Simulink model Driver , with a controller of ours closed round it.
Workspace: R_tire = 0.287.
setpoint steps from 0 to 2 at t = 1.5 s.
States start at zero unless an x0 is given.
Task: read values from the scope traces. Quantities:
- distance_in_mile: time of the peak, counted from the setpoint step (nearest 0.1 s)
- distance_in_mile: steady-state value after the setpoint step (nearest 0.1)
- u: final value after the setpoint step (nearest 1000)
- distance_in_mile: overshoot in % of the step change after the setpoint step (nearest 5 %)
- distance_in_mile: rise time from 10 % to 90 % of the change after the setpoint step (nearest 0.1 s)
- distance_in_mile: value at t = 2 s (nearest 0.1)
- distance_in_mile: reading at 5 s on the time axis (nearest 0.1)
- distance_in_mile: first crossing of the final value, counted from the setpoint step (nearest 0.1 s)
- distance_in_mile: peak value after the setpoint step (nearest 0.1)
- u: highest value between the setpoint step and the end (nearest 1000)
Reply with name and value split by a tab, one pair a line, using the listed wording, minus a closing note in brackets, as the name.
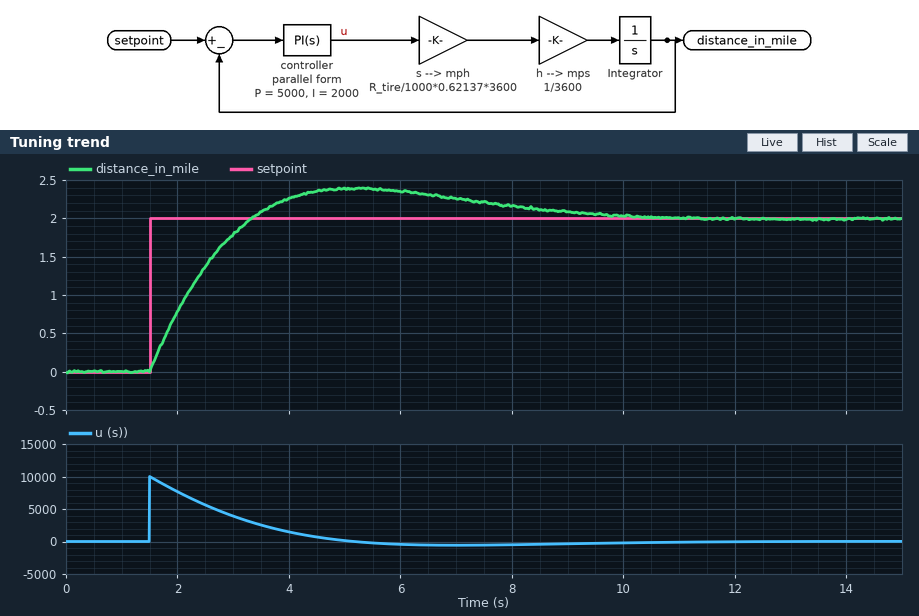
distance_in_mile: time of the peak, counted from the setpoint step	3.7 s
distance_in_mile: steady-state value after the setpoint step	2.0
u: final value after the setpoint step	0
distance_in_mile: overshoot in % of the step change after the setpoint step	20 %
distance_in_mile: rise time from 10 % to 90 % of the change after the setpoint step	1.4 s
distance_in_mile: value at t = 2 s	0.8
distance_in_mile: reading at 5 s on the time axis	2.4
distance_in_mile: first crossing of the final value, counted from the setpoint step	1.8 s
distance_in_mile: peak value after the setpoint step	2.4
u: highest value between the setpoint step and the end	10000
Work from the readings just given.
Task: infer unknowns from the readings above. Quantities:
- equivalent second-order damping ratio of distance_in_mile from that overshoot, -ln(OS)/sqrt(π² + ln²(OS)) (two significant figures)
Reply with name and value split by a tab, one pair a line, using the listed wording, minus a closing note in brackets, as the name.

equivalent second-order damping ratio of distance_in_mile from that overshoot, -ln(OS)/sqrt(π² + ln²(OS))	0.46
